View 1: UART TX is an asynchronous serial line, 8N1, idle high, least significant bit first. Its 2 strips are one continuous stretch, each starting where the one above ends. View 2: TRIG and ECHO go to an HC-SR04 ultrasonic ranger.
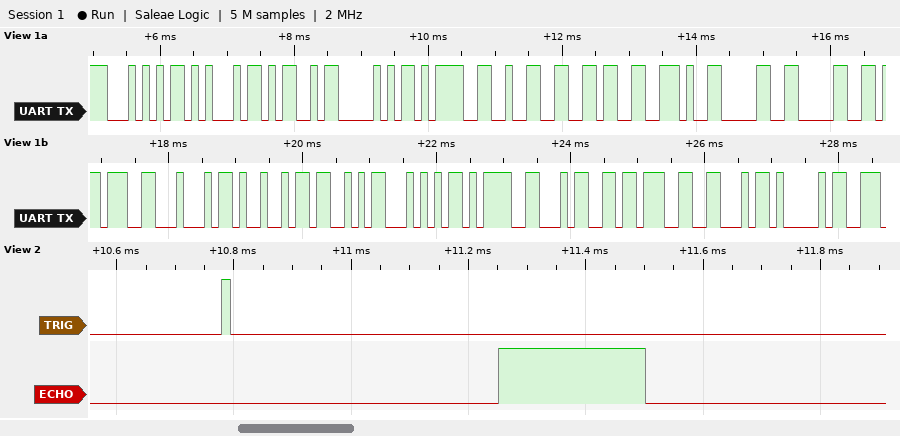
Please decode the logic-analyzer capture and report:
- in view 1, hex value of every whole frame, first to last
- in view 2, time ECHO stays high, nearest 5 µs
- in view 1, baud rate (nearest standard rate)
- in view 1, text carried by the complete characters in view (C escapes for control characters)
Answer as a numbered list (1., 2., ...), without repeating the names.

1. 54 45 4D 50 3D 32 36 2E 30 30 3B 44 49 53 54 3D 34 3B 46 41
2. 250 µs
3. 9600 baud
4. "TEMP=26.00;DIST=4;FA"
